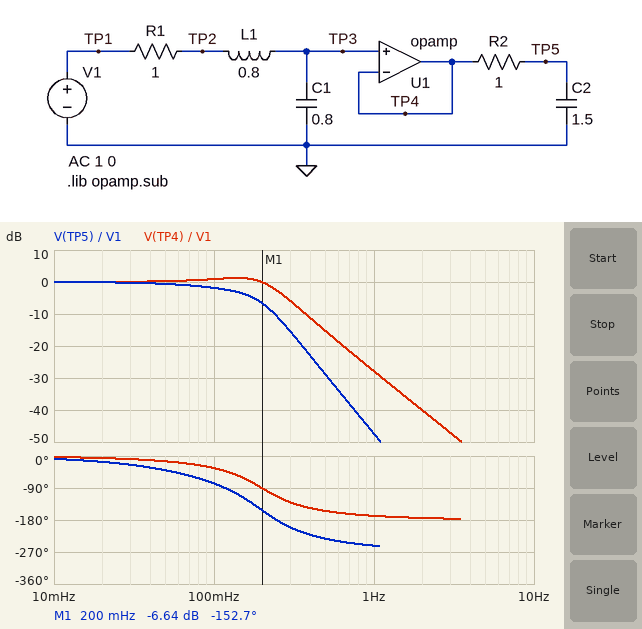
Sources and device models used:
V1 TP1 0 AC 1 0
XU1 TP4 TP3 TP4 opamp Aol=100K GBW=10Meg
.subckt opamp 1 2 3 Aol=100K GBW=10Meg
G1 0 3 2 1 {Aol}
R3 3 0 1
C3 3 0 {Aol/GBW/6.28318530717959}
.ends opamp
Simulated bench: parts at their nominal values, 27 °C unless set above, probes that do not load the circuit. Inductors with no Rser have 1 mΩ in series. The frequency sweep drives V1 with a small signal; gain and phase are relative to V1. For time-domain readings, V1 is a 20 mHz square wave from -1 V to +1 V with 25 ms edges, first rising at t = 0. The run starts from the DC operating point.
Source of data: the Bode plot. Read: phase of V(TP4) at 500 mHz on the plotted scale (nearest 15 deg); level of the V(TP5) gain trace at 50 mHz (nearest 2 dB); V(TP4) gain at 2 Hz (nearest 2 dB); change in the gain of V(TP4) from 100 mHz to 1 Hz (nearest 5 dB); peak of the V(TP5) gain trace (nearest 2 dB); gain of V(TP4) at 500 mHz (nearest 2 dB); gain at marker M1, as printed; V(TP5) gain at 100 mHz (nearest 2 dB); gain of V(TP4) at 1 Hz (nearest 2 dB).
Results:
-150 deg
0 dB
-40 dB
-30 dB
0 dB
-16 dB
-6.64 dB
-2 dB
-28 dB
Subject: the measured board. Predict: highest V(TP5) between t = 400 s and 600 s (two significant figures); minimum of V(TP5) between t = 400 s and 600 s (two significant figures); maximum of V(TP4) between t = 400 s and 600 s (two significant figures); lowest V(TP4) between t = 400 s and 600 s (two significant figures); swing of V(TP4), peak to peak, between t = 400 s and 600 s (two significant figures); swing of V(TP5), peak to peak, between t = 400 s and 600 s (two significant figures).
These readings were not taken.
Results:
1.0 V
-1.0 V
1.3 V
-1.3 V
2.7 V
2.0 V
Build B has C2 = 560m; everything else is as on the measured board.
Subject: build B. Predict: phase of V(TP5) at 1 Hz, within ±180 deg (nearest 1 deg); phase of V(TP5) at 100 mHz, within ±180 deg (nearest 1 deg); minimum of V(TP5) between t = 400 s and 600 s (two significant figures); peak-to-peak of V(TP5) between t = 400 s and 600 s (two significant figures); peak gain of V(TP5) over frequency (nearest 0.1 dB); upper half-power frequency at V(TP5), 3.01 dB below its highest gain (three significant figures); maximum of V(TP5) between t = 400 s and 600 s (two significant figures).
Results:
118 deg
-53 deg
-1.2 V
2.5 V
0.4 dB
212 mHz
1.2 V
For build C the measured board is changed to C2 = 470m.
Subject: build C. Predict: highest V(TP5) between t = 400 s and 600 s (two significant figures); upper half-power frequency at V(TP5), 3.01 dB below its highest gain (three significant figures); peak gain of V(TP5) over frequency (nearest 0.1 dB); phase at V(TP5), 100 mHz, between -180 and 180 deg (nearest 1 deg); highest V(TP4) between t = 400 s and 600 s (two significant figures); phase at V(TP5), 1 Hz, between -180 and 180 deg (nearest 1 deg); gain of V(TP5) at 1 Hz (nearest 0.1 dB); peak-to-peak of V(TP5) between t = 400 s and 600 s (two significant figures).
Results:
1.3 V
217 mHz
0.6 dB
-50 deg
1.3 V
120 deg
-37.8 dB
2.5 V
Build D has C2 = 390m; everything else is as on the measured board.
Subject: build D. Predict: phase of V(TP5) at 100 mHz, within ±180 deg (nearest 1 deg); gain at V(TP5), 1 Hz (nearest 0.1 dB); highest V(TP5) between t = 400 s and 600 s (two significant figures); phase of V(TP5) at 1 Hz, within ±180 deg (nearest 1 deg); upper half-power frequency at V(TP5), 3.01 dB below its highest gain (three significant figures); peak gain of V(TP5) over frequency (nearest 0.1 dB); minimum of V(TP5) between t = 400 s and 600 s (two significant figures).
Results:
-48 deg
-36.3 dB
1.3 V
124 deg
221 mHz
0.8 dB
-1.3 V
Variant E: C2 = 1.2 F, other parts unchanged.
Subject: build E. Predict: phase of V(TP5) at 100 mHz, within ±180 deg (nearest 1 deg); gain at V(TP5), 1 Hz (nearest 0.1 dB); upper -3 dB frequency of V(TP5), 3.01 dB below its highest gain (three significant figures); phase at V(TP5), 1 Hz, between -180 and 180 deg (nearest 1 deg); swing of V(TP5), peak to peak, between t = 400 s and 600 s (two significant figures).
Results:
-71 deg
-45.5 dB
165 mHz
109 deg
2.1 V
